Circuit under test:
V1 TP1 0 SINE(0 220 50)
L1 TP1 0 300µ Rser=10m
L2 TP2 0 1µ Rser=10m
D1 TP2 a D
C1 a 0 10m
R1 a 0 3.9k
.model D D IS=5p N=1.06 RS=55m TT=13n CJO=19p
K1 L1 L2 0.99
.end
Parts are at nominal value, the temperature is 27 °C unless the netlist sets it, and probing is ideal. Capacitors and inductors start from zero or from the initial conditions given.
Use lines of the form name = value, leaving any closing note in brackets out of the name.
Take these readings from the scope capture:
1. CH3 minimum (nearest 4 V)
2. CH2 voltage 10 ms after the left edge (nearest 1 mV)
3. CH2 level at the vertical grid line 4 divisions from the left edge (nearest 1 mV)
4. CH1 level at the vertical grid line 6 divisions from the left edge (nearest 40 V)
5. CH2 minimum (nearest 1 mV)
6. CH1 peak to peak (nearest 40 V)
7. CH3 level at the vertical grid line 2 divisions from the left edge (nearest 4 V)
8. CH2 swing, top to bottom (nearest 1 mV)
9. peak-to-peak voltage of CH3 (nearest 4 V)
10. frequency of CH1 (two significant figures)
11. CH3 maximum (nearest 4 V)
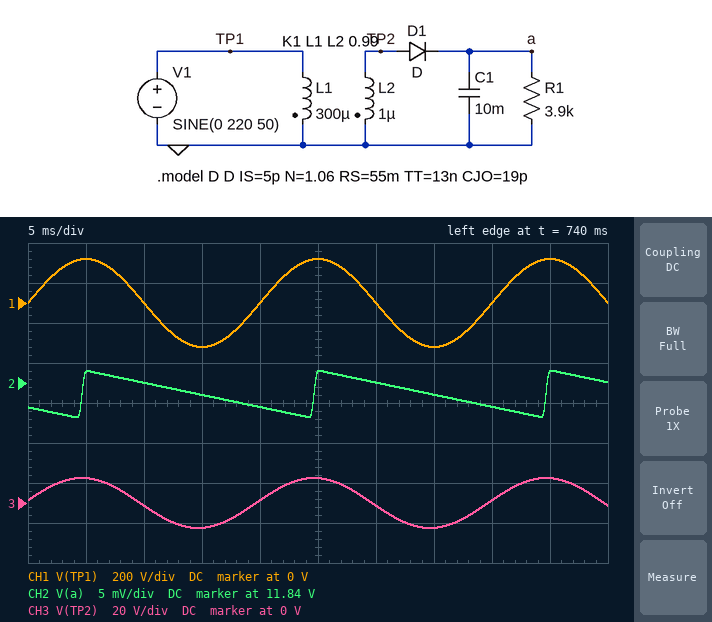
CH3 minimum = -12 V
CH2 voltage 10 ms after the left edge = 11.835 V
CH2 level at the vertical grid line 4 divisions from the left edge = 11.832 V
CH1 level at the vertical grid line 6 divisions from the left edge = 0 V
CH2 minimum = 11.831 V
CH1 peak to peak = 440 V
CH3 level at the vertical grid line 2 divisions from the left edge = 0 V
CH2 swing, top to bottom = 6 mV
peak-to-peak voltage of CH3 = 24 V
frequency of CH1 = 50 Hz
CH3 maximum = 12 V
